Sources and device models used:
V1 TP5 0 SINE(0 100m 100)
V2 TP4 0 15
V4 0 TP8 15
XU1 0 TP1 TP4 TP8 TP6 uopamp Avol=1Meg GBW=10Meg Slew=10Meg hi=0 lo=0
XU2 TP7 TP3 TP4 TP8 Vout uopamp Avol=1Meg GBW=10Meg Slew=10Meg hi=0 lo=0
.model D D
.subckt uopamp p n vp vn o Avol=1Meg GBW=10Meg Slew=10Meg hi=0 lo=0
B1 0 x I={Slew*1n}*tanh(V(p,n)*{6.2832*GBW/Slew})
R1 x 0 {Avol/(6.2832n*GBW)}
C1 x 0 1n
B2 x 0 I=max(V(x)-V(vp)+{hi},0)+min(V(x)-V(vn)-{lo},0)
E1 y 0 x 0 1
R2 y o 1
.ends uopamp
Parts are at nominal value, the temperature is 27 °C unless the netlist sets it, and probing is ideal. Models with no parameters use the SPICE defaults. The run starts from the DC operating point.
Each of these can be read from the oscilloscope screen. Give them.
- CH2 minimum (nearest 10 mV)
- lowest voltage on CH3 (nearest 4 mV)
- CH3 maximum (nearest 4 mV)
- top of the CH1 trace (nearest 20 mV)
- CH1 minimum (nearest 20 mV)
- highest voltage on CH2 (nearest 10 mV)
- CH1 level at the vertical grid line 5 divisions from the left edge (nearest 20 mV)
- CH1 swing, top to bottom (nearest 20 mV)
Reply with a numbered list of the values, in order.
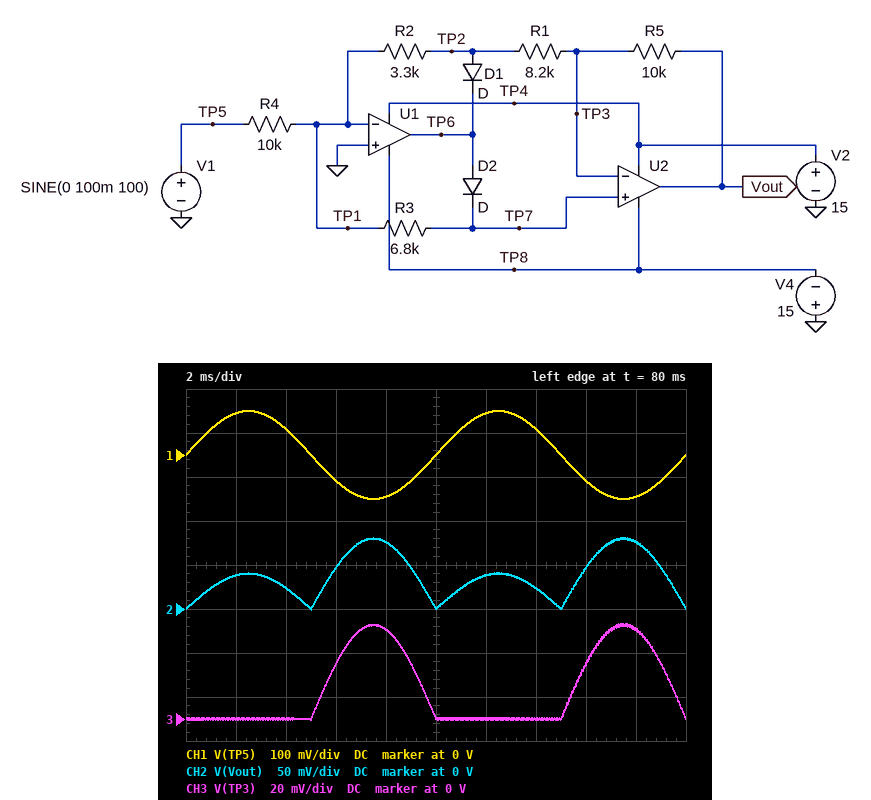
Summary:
1. 0 V
2. 0 V
3. 44 mV
4. 100 mV
5. -100 mV
6. 80 mV
7. 0 V
8. 200 mV
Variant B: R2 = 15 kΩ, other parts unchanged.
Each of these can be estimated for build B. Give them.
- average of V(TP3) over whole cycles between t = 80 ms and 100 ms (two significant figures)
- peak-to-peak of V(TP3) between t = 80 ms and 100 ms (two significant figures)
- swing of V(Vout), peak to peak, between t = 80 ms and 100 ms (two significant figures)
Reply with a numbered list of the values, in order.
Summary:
1. 17 mV
2. 54 mV
3. 180 mV
